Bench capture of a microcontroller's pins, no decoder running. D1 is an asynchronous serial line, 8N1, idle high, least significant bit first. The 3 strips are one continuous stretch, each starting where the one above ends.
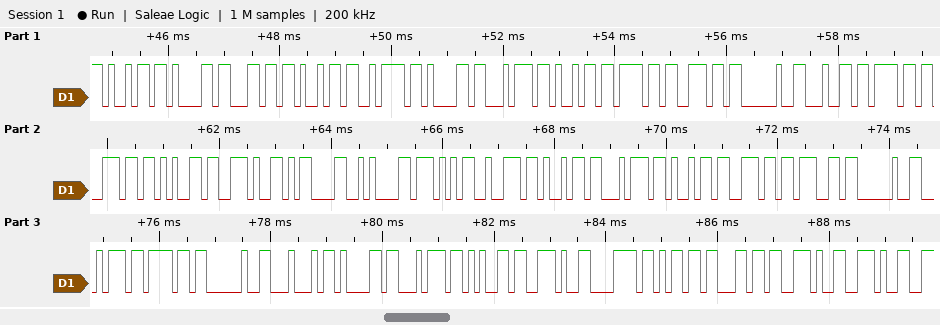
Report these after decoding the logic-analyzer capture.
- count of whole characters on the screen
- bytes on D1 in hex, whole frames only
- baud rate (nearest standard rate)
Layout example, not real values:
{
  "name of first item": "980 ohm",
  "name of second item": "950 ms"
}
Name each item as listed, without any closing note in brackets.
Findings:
{
  "count of whole characters on the screen": "39",
  "bytes on D1 in hex, whole frames only": "69 61 6C 69 7A 61 74 69 6F 6E 20 64 6F 6E 65 2E 0D 0A 57 72 69 74 69 6E 67 20 74 6F 20 44 61 74 65 2E 78 6D 6C 2E 2E",
  "baud rate": "9600 baud"
}
